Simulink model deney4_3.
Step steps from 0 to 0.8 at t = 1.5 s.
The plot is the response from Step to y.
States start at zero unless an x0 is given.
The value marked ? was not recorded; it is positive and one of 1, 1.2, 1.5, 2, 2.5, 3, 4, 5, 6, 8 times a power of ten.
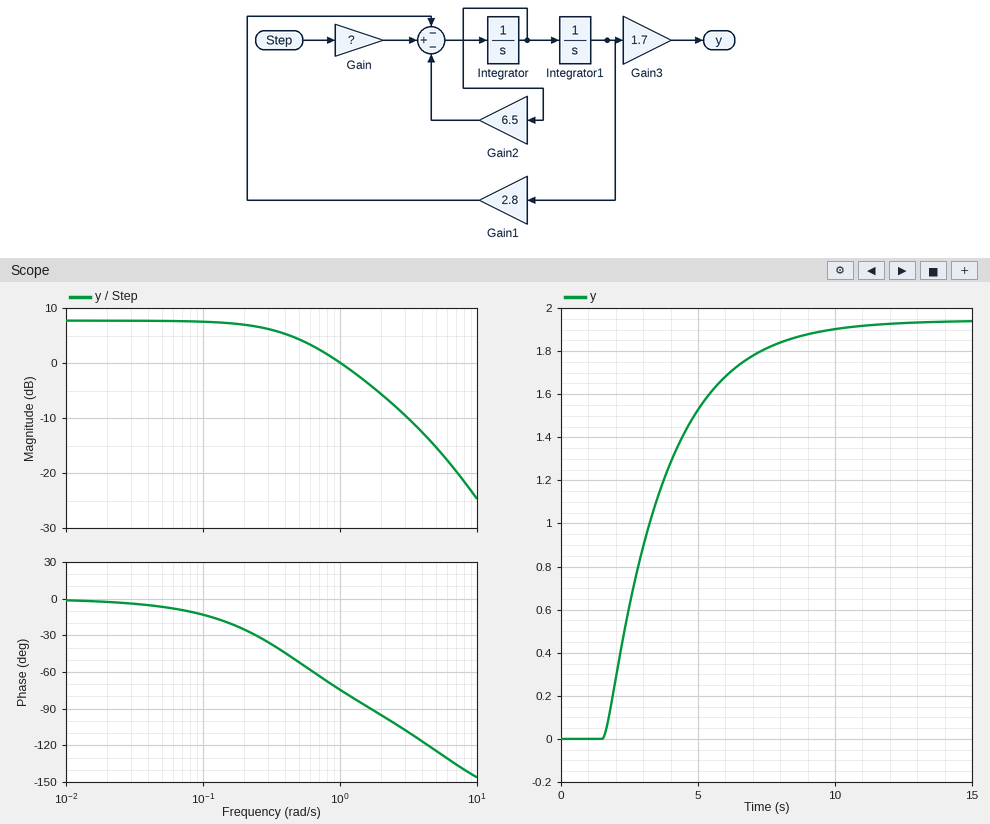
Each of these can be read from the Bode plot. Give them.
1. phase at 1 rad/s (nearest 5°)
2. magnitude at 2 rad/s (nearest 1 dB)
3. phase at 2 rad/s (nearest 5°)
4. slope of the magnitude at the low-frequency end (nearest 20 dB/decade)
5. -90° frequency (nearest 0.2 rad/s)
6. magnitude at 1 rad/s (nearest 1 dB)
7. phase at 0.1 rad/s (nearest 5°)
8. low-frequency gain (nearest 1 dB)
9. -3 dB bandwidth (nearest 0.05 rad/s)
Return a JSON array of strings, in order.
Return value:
["-75°", "-6 dB", "-95°", "0 dB/decade", "1.6 rad/s", "0 dB", "-15°", "8 dB", "0.45 rad/s"]
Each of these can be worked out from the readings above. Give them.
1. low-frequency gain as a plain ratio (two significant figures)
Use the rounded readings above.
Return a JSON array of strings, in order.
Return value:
["2.5"]
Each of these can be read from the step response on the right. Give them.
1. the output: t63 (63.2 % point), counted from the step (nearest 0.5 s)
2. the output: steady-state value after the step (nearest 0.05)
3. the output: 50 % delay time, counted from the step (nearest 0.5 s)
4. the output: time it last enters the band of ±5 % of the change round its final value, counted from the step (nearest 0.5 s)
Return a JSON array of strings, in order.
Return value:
["2.5 s", "1.95", "1.5 s", "6.5 s"]
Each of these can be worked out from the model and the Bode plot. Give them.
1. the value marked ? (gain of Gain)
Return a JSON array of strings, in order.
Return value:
["4"]
